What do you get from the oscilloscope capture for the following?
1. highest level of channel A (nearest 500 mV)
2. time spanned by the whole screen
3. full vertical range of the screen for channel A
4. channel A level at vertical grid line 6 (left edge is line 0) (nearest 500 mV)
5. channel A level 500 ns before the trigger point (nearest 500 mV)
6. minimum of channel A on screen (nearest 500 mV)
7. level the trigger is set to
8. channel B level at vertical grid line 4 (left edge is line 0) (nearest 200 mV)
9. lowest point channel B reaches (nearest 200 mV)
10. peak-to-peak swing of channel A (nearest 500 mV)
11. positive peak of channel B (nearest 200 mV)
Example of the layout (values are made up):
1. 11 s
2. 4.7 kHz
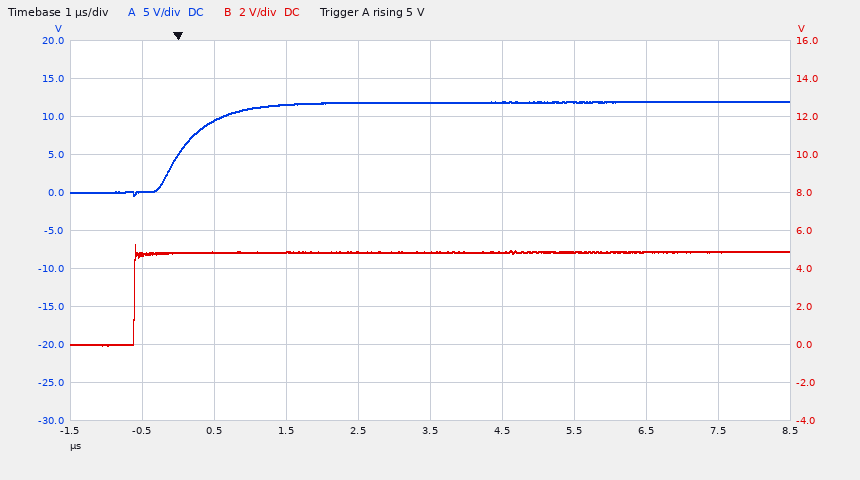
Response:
1. 12.0 V
2. 10 µs
3. 50 V
4. 12.0 V
5. 0.0 V
6. -500 mV
7. 5 V
8. 4.8 V
9. 0.0 V
10. 12.5 V
11. 5.2 V
